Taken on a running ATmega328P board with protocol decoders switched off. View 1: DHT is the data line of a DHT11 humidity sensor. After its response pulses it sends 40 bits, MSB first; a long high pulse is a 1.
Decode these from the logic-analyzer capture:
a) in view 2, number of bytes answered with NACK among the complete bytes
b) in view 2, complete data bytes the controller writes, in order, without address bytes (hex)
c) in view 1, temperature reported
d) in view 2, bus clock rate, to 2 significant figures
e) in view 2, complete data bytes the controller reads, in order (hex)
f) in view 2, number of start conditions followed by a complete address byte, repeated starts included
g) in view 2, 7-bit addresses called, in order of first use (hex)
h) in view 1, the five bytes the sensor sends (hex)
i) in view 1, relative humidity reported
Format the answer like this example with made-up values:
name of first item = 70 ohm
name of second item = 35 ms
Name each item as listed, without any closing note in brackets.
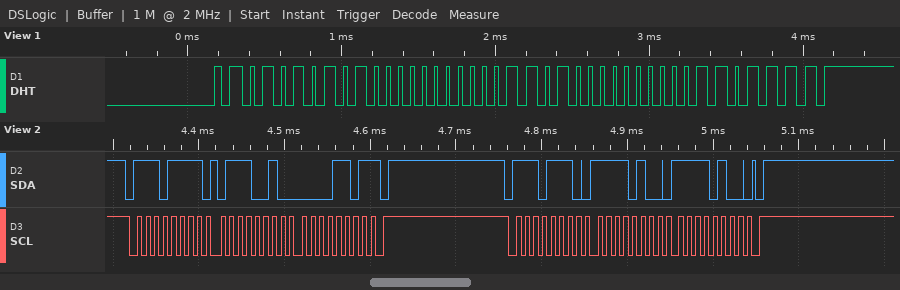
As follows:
in view 2, number of bytes answered with NACK among the complete bytes = 1
in view 2, complete data bytes the controller writes, in order, without address bytes = F4 F4
in view 1, temperature reported = 26.0 °C
in view 2, bus clock rate, to 2 significant figures = 100 kHz
in view 2, complete data bytes the controller reads, in order = 72 0D
in view 2, number of start conditions followed by a complete address byte, repeated starts included = 2
in view 2, 7-bit addresses called, in order of first use = 0x77
in view 1, the five bytes the sensor sends = 55 00 1A 00 6F
in view 1, relative humidity reported = 85 %
